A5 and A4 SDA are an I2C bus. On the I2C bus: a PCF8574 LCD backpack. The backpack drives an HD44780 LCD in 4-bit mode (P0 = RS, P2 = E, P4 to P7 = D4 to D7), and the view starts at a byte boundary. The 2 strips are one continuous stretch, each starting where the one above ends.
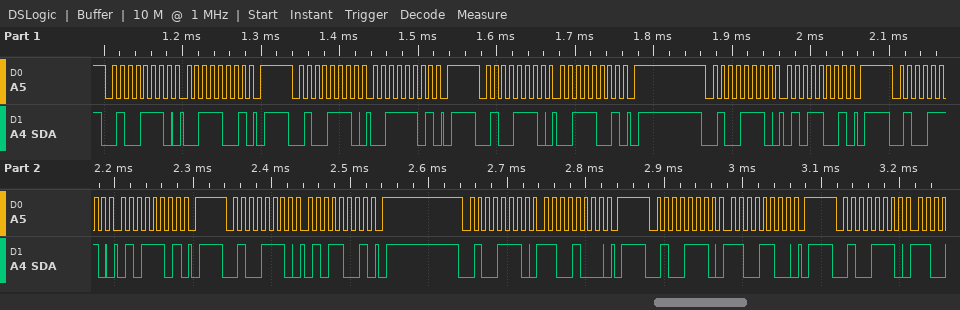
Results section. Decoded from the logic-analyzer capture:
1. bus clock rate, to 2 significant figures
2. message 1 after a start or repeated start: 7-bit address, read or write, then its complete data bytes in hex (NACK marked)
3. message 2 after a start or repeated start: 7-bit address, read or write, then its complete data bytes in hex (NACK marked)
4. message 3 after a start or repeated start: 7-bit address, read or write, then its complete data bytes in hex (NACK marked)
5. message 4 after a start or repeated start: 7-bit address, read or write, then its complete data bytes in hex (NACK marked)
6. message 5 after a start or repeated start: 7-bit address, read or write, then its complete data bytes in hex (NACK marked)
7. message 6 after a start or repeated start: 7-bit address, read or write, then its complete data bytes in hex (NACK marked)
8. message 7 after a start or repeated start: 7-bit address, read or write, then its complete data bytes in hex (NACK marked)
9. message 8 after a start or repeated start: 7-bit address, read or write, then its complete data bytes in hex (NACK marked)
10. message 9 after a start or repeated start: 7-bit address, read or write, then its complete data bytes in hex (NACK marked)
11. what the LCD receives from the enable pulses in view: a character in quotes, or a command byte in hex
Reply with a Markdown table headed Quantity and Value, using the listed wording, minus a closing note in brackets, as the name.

| Quantity | Value |
|---|---|
| bus clock rate, to 2 significant figures | 100 kHz |
| message 1 after a start or repeated start: 7-bit address, read or write, then its complete data bytes in hex | 0x27 write: 39 |
| message 2 after a start or repeated start: 7-bit address, read or write, then its complete data bytes in hex | 0x27 write: 3D |
| message 3 after a start or repeated start: 7-bit address, read or write, then its complete data bytes in hex | 0x27 write: 39 |
| message 4 after a start or repeated start: 7-bit address, read or write, then its complete data bytes in hex | 0x27 write: 59 |
| message 5 after a start or repeated start: 7-bit address, read or write, then its complete data bytes in hex | 0x27 write: 5D |
| message 6 after a start or repeated start: 7-bit address, read or write, then its complete data bytes in hex | 0x27 write: 59 |
| message 7 after a start or repeated start: 7-bit address, read or write, then its complete data bytes in hex | 0x27 write: C8 |
| message 8 after a start or repeated start: 7-bit address, read or write, then its complete data bytes in hex | 0x27 write: CC |
| message 9 after a start or repeated start: 7-bit address, read or write, then its complete data bytes in hex | 0x27 write |
| what the LCD receives from the enable pulses in view: a character in quotes, or a command byte in hex | '5' |
